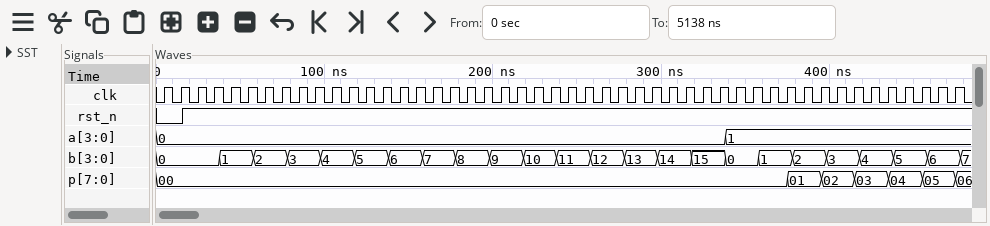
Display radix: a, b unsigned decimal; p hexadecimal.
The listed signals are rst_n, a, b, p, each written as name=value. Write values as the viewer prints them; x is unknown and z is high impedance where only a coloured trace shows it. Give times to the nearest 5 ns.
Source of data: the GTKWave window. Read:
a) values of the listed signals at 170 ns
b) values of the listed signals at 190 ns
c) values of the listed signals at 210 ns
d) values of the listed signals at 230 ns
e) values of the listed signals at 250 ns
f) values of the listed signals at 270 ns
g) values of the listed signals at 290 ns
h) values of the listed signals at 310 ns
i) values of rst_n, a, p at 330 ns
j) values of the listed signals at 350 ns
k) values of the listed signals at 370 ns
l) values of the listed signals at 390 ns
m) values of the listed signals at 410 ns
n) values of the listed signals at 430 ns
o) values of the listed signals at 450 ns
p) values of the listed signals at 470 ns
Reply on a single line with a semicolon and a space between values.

rst_n=1, a=0, b=7, p=00; rst_n=1, a=0, b=8, p=00; rst_n=1, a=0, b=9, p=00; rst_n=1, a=0, b=10, p=00; rst_n=1, a=0, b=11, p=00; rst_n=1, a=0, b=12, p=00; rst_n=1, a=0, b=13, p=00; rst_n=1, a=0, b=14, p=00; rst_n=1, a=0, p=00; rst_n=1, a=1, b=0, p=00; rst_n=1, a=1, b=1, p=00; rst_n=1, a=1, b=2, p=01; rst_n=1, a=1, b=3, p=02; rst_n=1, a=1, b=4, p=03; rst_n=1, a=1, b=5, p=04; rst_n=1, a=1, b=6, p=05
